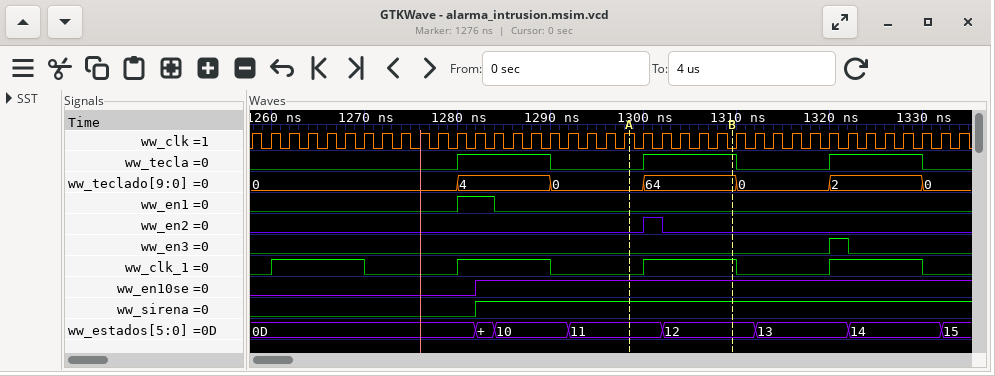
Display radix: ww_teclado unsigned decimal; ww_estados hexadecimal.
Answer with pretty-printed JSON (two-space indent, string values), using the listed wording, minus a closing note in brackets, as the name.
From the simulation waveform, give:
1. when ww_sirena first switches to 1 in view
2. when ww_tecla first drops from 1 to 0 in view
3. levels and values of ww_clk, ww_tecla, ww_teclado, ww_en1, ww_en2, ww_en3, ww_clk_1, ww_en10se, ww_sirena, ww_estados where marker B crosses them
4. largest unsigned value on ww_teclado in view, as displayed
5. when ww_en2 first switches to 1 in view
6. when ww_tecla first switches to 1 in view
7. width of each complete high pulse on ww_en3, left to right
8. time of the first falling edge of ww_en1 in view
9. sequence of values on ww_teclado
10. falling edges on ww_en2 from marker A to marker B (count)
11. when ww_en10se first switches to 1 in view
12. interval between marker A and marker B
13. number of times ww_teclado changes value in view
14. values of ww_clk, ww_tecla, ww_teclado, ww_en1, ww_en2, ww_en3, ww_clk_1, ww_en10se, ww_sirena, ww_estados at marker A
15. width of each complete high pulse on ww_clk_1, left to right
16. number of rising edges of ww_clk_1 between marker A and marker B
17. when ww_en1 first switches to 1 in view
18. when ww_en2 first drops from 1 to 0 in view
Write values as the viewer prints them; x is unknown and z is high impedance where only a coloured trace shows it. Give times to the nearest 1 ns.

{
  "when ww_sirena first switches to 1 in view": "1282 ns",
  "when ww_tecla first drops from 1 to 0 in view": "1290 ns",
  "levels and values of ww_clk, ww_tecla, ww_teclado, ww_en1, ww_en2, ww_en3, ww_clk_1, ww_en10se, ww_sirena, ww_estados where marker B crosses them": "ww_clk=0, ww_tecla=1, ww_teclado=64, ww_en1=0, ww_en2=0, ww_en3=0, ww_clk_1=1, ww_en10se=1, ww_sirena=1, ww_estados=12",
  "largest unsigned value on ww_teclado in view, as displayed": "64",
  "when ww_en2 first switches to 1 in view": "1300 ns",
  "when ww_tecla first switches to 1 in view": "1280 ns",
  "width of each complete high pulse on ww_en3, left to right": "2 ns",
  "time of the first falling edge of ww_en1 in view": "1284 ns",
  "sequence of values on ww_teclado": "0, 4, 0, 64, 0, 2, 0",
  "falling edges on ww_en2 from marker A to marker B": "1",
  "when ww_en10se first switches to 1 in view": "1282 ns",
  "interval between marker A and marker B": "11 ns",
  "number of times ww_teclado changes value in view": "6",
  "values of ww_clk, ww_tecla, ww_teclado, ww_en1, ww_en2, ww_en3, ww_clk_1, ww_en10se, ww_sirena, ww_estados at marker A": "ww_clk=1, ww_tecla=0, ww_teclado=0, ww_en1=0, ww_en2=0, ww_en3=0, ww_clk_1=0, ww_en10se=1, ww_sirena=1, ww_estados=11",
  "width of each complete high pulse on ww_clk_1, left to right": "10 ns, 10 ns, 10 ns, 10 ns",
  "number of rising edges of ww_clk_1 between marker A and marker B": "1",
  "when ww_en1 first switches to 1 in view": "1280 ns",
  "when ww_en2 first drops from 1 to 0 in view": "1302 ns"
}
